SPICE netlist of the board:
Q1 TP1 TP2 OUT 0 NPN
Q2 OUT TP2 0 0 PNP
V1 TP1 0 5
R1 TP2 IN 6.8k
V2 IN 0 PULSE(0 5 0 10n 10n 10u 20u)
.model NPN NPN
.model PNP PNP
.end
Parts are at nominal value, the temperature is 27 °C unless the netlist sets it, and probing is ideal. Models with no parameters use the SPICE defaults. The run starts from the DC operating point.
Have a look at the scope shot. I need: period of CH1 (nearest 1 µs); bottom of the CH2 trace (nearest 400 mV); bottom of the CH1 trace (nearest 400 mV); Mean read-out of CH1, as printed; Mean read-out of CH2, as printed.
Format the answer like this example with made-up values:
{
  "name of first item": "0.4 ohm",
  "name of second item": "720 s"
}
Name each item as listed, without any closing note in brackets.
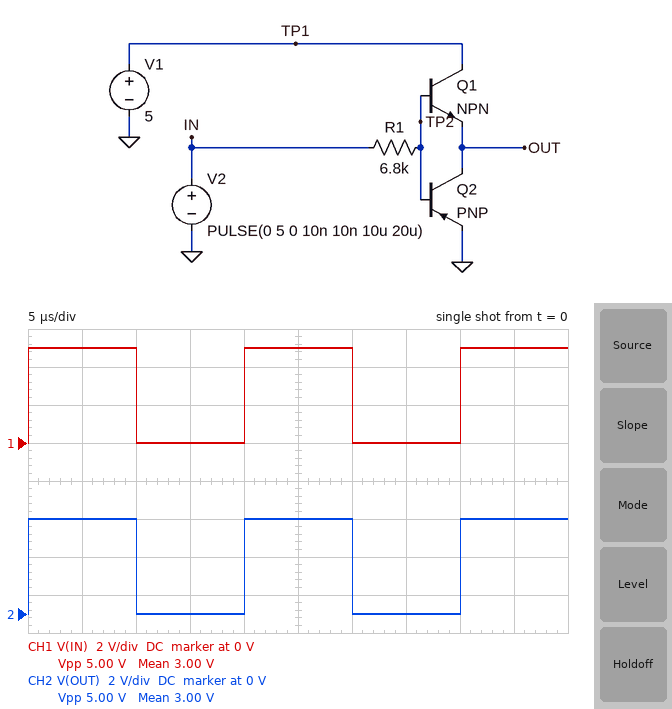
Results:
{
  "period of CH1": "20 µs",
  "bottom of the CH2 trace": "0 V",
  "bottom of the CH1 trace": "0 V",
  "Mean read-out of CH1, as printed": "3.00 V",
  "Mean read-out of CH2, as printed": "3.00 V"
}
